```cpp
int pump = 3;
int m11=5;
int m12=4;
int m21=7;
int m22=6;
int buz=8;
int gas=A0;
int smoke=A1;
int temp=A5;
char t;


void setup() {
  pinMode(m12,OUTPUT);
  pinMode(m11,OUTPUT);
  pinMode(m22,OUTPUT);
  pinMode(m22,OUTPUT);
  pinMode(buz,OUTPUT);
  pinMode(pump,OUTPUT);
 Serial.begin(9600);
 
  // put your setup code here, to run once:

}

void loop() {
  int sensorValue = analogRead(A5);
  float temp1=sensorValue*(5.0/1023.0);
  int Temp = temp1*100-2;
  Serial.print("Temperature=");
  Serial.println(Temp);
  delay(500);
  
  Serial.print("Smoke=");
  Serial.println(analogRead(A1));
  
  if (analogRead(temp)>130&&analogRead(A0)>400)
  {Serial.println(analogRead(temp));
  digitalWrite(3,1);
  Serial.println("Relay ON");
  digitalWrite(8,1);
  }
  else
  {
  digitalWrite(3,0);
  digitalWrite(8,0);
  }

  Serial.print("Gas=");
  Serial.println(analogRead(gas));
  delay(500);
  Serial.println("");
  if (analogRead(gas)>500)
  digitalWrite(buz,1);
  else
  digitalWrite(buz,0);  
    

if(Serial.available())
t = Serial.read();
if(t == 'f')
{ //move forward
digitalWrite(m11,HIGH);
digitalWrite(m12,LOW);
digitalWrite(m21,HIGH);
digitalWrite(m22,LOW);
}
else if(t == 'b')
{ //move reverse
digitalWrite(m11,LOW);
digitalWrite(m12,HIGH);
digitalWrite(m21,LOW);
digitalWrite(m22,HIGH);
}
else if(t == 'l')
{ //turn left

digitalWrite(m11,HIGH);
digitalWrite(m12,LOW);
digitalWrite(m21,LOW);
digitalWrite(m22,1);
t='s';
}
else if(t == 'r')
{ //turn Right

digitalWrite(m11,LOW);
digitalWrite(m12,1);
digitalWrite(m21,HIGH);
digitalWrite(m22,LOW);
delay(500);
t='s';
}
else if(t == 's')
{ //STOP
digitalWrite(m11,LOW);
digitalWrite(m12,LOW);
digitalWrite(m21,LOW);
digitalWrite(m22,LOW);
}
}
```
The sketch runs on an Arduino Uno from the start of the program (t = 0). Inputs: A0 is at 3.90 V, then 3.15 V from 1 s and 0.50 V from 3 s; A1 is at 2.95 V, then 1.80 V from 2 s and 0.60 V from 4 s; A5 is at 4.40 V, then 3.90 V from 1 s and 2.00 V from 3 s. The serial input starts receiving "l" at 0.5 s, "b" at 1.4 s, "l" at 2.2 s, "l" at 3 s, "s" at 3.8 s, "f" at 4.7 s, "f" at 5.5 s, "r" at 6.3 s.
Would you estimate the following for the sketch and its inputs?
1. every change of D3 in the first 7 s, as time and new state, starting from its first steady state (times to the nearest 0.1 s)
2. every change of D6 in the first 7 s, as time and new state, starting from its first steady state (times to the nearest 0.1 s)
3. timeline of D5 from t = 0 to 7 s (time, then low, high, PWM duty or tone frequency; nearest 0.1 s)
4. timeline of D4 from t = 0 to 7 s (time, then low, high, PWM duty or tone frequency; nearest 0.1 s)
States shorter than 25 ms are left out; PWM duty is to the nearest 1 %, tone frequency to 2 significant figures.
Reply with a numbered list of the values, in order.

1. 0 s low; 0.5 s high; 3.5 s low
2. 0 s low; 1 s high; 5 s low
3. 0 s low; 1 s high; 2 s low; 3 s high; 5 s low; 6 s high
4. 0 s low; 2 s high; 3 s low
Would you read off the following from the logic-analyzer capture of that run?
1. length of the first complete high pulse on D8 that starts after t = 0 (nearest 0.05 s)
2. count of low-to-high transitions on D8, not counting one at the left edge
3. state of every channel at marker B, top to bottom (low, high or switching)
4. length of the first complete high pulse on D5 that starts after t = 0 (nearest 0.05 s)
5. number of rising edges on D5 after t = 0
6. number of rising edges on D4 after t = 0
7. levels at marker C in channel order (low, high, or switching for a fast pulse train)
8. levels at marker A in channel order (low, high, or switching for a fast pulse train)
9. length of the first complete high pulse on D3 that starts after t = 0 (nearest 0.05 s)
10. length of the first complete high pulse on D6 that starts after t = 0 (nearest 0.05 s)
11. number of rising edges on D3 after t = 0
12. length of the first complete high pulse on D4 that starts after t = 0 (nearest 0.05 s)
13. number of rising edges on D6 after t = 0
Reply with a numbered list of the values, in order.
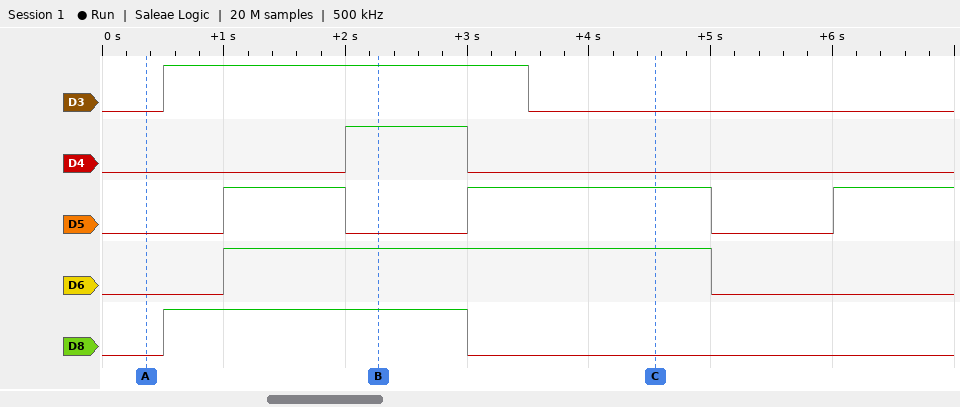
1. 2.50 s
2. 1
3. D3 high, D4 high, D5 low, D6 high, D8 high
4. 1.00 s
5. 3
6. 1
7. D3 low, D4 low, D5 high, D6 high, D8 low
8. D3 low, D4 low, D5 low, D6 low, D8 low
9. 3.00 s
10. 4.00 s
11. 1
12. 1.00 s
13. 1
